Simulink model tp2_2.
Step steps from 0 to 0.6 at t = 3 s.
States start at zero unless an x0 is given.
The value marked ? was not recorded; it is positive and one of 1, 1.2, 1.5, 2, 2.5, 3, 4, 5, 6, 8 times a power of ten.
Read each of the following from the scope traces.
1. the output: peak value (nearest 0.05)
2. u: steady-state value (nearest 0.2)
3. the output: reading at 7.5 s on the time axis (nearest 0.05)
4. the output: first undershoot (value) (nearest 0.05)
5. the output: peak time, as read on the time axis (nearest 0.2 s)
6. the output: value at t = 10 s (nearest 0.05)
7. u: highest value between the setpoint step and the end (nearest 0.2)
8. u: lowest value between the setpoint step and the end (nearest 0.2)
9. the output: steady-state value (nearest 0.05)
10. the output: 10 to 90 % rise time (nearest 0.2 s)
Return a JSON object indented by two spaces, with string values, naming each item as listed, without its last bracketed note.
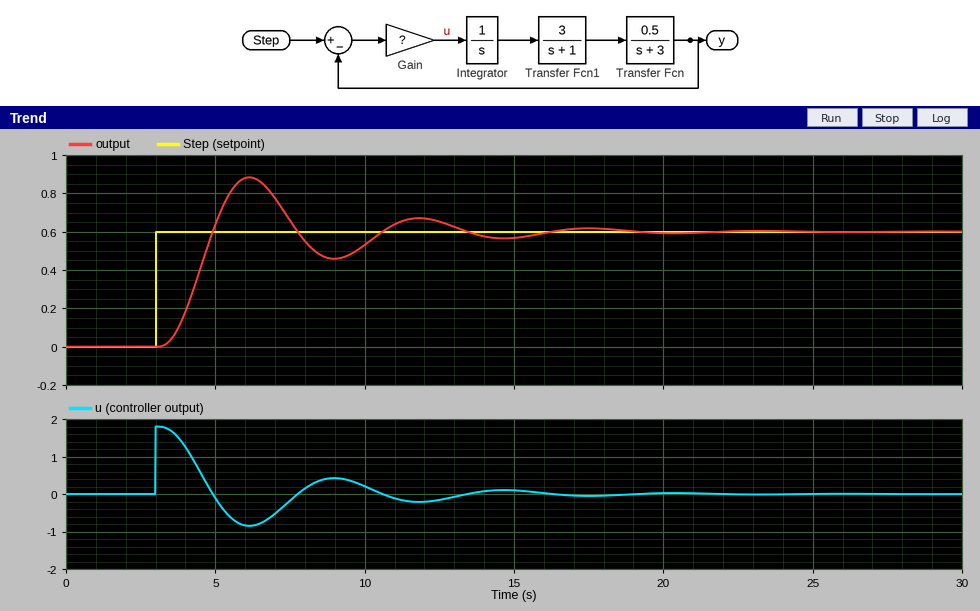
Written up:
{
  "the output: peak value": "0.90",
  "u: steady-state value": "0.0",
  "the output: reading at 7.5 s on the time axis": "0.65",
  "the output: first undershoot (value)": "0.45",
  "the output: peak time, as read on the time axis": "6.2 s",
  "the output: value at t = 10 s": "0.55",
  "u: highest value between the setpoint step and the end": "1.8",
  "u: lowest value between the setpoint step and the end": "-0.8",
  "the output: steady-state value": "0.60",
  "the output: 10 to 90 % rise time": "1.2 s"
}
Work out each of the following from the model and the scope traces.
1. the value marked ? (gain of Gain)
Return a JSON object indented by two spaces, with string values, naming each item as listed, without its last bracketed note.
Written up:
{
  "the value marked ?": "3"
}
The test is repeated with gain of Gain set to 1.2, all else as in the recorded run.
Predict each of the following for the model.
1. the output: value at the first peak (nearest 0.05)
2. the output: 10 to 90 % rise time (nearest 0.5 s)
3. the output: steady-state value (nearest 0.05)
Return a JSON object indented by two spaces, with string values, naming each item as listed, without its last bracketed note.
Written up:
{
  "the output: value at the first peak": "0.70",
  "the output: 10 to 90 % rise time": "2.5 s",
  "the output: steady-state value": "0.60"
}
